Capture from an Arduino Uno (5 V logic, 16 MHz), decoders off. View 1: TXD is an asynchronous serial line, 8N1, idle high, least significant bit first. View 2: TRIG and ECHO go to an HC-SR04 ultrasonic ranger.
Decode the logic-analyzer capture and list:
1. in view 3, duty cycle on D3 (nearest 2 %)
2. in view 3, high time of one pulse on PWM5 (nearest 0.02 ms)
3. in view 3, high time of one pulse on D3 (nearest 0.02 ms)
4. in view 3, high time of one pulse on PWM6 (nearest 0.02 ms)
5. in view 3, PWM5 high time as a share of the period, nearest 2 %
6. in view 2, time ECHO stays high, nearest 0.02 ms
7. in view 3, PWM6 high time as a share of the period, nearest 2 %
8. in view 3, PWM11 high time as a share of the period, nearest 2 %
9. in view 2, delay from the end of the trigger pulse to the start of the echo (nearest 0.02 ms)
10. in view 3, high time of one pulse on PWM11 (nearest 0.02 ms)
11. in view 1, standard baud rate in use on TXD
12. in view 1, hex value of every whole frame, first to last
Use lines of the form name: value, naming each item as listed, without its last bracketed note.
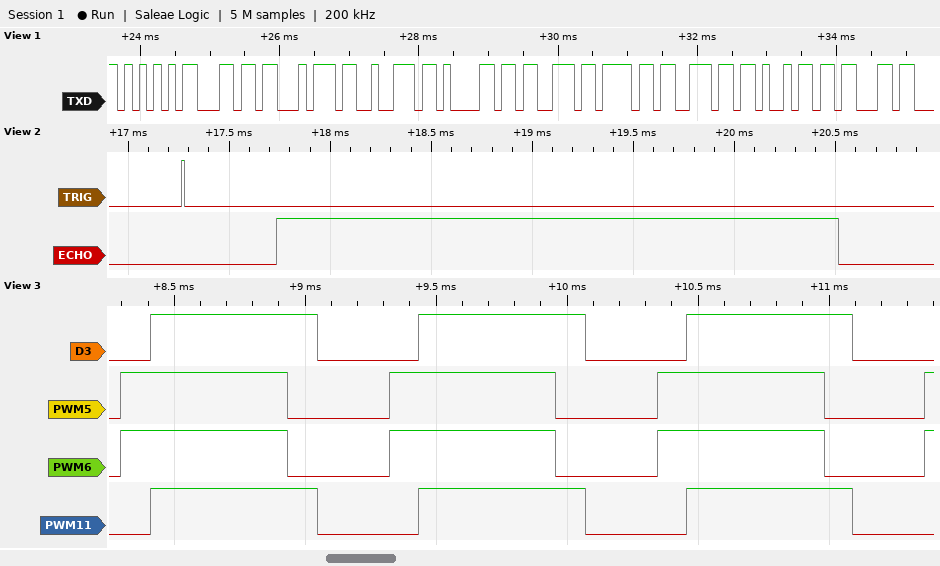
in view 3, duty cycle on D3: 62 %
in view 3, high time of one pulse on PWM5: 0.64 ms
in view 3, high time of one pulse on D3: 0.64 ms
in view 3, high time of one pulse on PWM6: 0.64 ms
in view 3, PWM5 high time as a share of the period, nearest 2 %: 62 %
in view 2, time ECHO stays high, nearest 0.02 ms: 2.78 ms
in view 3, PWM6 high time as a share of the period, nearest 2 %: 62 %
in view 3, PWM11 high time as a share of the period, nearest 2 %: 62 %
in view 2, delay from the end of the trigger pulse to the start of the echo: 0.46 ms
in view 3, high time of one pulse on PWM11: 0.64 ms
in view 1, standard baud rate in use on TXD: 9600 baud
in view 1, hex value of every whole frame, first to last: 0x55 0x6C 0x74 0x72 0x61 0x73 0x6F 0x6E 0x69 0x63
